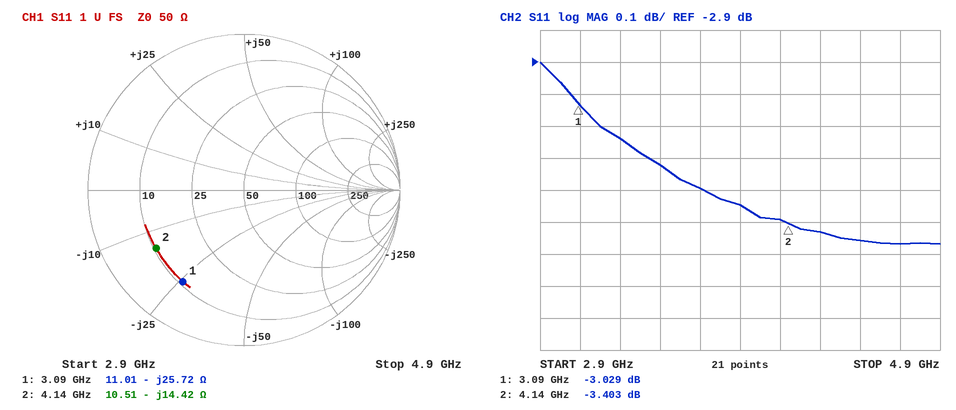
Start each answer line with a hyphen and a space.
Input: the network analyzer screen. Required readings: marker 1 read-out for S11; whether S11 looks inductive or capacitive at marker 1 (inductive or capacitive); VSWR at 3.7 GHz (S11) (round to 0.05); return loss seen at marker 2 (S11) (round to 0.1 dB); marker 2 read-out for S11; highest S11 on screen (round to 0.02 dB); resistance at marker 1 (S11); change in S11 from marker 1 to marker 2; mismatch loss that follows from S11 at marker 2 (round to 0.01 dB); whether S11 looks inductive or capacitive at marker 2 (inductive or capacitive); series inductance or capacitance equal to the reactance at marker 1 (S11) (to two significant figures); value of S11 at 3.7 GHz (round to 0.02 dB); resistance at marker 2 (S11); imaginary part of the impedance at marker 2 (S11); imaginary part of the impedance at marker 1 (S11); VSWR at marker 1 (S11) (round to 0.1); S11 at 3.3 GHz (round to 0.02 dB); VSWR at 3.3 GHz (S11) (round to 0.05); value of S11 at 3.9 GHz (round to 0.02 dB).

- -3.029 dB
- capacitive
- 5.35
- 3.4 dB
- -3.403 dB
- -2.90 dB
- 11.01 Ω
- -0.374 dB
- 2.65 dB
- capacitive
- 2.0 pF
- -3.30 dB
- 10.51 Ω
- -14.42 Ω
- -25.72 Ω
- 5.8
- -3.14 dB
- 5.60
- -3.34 dB
